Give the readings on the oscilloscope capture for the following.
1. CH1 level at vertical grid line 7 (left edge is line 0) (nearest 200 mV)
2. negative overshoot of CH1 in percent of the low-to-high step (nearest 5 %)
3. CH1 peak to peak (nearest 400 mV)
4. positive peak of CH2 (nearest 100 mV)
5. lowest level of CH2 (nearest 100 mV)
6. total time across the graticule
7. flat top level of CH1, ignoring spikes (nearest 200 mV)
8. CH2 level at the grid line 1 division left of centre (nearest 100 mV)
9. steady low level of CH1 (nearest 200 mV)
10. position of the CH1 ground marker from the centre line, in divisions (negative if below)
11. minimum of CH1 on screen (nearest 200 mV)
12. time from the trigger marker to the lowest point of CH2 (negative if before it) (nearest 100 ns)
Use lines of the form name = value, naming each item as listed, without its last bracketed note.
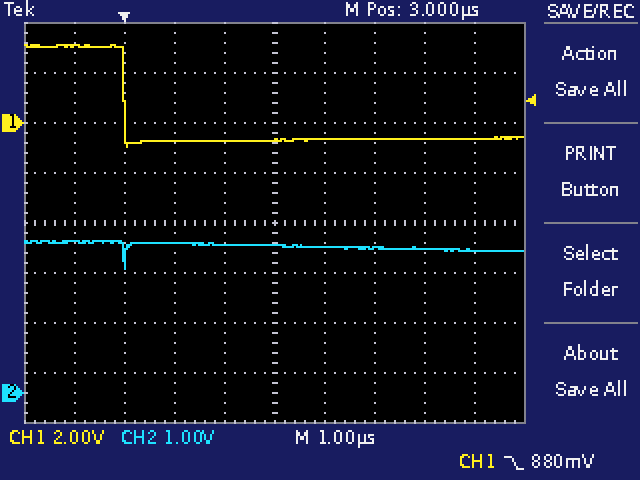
CH1 level at vertical grid line 7 (left edge is line 0) = -600 mV
negative overshoot of CH1 in percent of the low-to-high step = 10 %
CH1 peak to peak = 4.0 V
positive peak of CH2 = 3.0 V
lowest level of CH2 = 2.5 V
total time across the graticule = 10 µs
flat top level of CH1, ignoring spikes = 3.0 V
CH2 level at the grid line 1 division left of centre = 3.0 V
steady low level of CH1 = -600 mV
position of the CH1 ground marker from the centre line, in divisions = +2.0 div
minimum of CH1 on screen = -1.0 V
time from the trigger marker to the lowest point of CH2 (negative if before it) = 0.0 µs
